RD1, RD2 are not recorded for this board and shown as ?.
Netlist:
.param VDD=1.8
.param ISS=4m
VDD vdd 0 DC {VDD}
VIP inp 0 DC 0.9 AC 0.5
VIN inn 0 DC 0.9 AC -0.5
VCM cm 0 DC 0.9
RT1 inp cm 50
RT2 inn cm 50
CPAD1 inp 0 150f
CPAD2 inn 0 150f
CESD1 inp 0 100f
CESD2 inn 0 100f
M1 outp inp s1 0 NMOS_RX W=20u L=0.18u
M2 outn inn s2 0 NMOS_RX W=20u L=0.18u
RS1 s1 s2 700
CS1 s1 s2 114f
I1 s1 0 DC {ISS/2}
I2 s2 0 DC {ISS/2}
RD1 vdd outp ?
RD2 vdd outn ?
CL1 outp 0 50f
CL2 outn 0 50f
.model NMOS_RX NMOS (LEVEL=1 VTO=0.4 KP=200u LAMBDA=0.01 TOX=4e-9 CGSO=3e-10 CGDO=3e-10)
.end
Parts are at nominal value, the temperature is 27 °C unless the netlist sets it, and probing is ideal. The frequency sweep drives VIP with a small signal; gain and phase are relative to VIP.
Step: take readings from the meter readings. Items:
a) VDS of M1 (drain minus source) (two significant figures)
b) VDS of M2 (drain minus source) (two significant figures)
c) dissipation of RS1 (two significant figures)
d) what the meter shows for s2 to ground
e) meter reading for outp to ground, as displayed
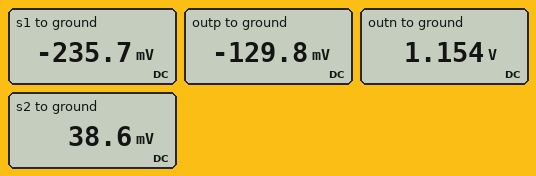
110 mV
1.1 V
110 µW
38.6 mV
-129.8 mV
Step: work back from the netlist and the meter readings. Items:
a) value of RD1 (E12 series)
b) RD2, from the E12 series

1.2 kΩ
270 Ω
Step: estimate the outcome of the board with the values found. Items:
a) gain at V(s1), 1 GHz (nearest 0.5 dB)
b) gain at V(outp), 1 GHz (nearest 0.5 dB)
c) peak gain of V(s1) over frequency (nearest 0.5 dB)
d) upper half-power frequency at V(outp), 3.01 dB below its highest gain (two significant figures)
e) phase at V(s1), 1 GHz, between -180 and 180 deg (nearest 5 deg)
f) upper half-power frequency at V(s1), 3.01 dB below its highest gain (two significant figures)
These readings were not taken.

-14.0 dB
-8.5 dB
-13.0 dB
2.5 GHz
145 deg
2.2 GHz
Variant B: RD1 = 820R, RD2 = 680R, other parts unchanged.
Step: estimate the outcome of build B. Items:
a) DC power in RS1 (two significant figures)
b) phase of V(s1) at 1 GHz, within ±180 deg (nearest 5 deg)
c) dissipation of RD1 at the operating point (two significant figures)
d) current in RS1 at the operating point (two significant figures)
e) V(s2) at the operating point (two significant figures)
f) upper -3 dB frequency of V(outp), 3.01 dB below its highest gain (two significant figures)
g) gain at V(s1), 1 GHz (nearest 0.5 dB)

4.1 µW
15 deg
3.0 mW
77 µA
54 mV
5.4 GHz
-15.0 dB
